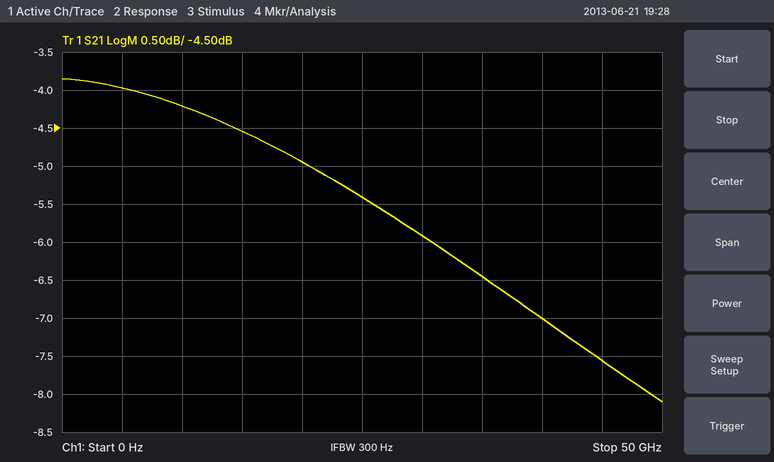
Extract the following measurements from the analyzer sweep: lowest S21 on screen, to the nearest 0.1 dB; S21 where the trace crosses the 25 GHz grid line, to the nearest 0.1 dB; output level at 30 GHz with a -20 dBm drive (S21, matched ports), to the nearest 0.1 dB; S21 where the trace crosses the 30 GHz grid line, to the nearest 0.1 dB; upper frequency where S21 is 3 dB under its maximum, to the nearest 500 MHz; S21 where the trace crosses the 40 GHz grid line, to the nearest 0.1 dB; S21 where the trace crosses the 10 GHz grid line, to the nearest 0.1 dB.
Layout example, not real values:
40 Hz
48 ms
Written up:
-8.1 dB
-5.4 dB
-25.9 dBm
-5.9 dB
38.5 GHz
-7.0 dB
-4.2 dB
